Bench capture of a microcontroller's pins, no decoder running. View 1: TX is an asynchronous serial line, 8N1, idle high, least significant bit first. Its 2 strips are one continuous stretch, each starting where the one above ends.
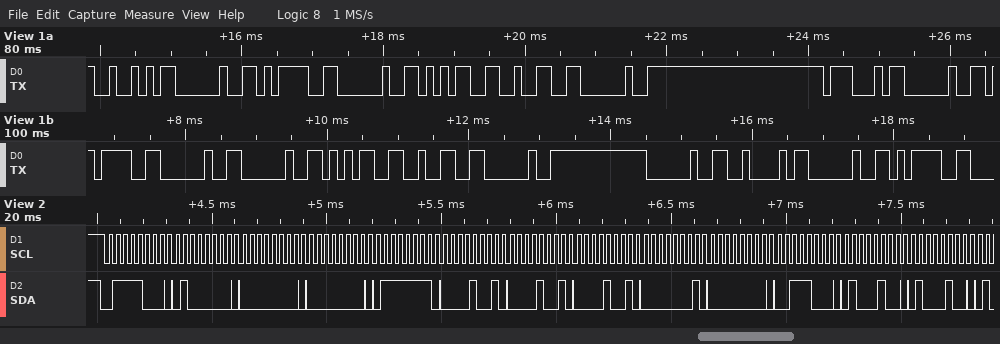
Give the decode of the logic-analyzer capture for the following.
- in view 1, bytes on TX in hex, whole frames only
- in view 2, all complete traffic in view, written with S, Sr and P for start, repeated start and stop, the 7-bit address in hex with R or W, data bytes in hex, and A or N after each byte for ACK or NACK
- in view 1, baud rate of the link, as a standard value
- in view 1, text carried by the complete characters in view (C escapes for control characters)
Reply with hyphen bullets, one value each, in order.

- 52 20 3D 20 35 32 20 47 20 3D 20 20 35 32 20 20 42 20 3D
- S 3CW A 40 A 00 A 00 A 7F A 09 A 09 A 09 A 01 A 00 A 38 A 44 A 44 A
- 9600 baud
- "R = 52 G =  52  B ="
